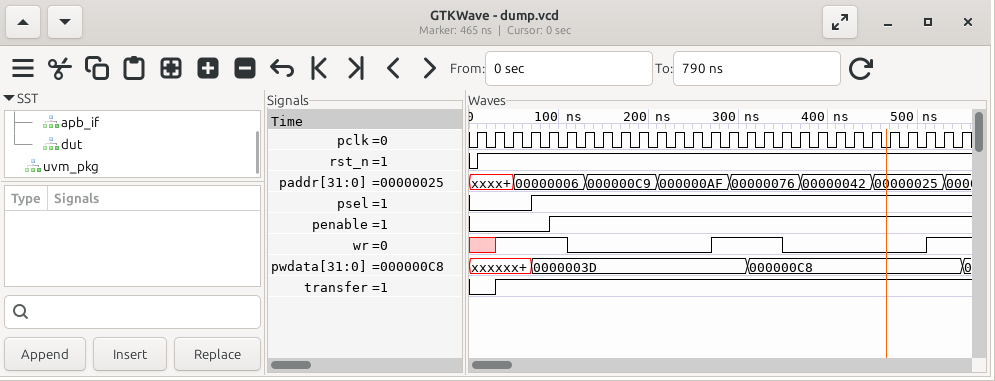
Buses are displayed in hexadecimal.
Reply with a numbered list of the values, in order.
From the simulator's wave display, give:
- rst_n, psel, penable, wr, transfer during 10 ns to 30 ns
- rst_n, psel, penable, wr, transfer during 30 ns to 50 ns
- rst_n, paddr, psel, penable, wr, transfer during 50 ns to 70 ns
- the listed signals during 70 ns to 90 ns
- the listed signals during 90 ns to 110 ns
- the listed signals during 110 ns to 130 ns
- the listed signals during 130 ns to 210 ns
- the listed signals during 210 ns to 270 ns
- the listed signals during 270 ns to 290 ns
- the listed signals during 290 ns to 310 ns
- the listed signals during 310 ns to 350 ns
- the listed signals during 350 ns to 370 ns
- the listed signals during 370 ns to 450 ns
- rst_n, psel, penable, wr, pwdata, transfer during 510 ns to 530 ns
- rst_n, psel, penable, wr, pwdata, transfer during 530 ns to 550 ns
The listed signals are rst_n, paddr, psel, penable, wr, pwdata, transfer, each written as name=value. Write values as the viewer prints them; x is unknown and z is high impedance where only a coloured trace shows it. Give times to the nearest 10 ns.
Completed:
1. rst_n=1, psel=0, penable=0, wr=x, transfer=0
2. rst_n=1, psel=0, penable=0, wr=1, transfer=1
3. rst_n=1, paddr=00000006, psel=0, penable=0, wr=1, transfer=1
4. rst_n=1, paddr=00000006, psel=1, penable=0, wr=1, pwdata=0000003D, transfer=1
5. rst_n=1, paddr=00000006, psel=1, penable=1, wr=1, pwdata=0000003D, transfer=1
6. rst_n=1, paddr=00000006, psel=1, penable=1, wr=0, pwdata=0000003D, transfer=1
7. rst_n=1, paddr=000000C9, psel=1, penable=1, wr=0, pwdata=0000003D, transfer=1
8. rst_n=1, paddr=000000AF, psel=1, penable=1, wr=0, pwdata=0000003D, transfer=1
9. rst_n=1, paddr=000000AF, psel=1, penable=1, wr=1, pwdata=0000003D, transfer=1
10. rst_n=1, paddr=00000076, psel=1, penable=1, wr=1, pwdata=0000003D, transfer=1
11. rst_n=1, paddr=00000076, psel=1, penable=1, wr=1, pwdata=000000C8, transfer=1
12. rst_n=1, paddr=00000076, psel=1, penable=1, wr=0, pwdata=000000C8, transfer=1
13. rst_n=1, paddr=00000042, psel=1, penable=1, wr=0, pwdata=000000C8, transfer=1
14. rst_n=1, psel=1, penable=1, wr=1, pwdata=000000C8, transfer=1
15. rst_n=1, psel=1, penable=1, wr=1, pwdata=000000C8, transfer=1
